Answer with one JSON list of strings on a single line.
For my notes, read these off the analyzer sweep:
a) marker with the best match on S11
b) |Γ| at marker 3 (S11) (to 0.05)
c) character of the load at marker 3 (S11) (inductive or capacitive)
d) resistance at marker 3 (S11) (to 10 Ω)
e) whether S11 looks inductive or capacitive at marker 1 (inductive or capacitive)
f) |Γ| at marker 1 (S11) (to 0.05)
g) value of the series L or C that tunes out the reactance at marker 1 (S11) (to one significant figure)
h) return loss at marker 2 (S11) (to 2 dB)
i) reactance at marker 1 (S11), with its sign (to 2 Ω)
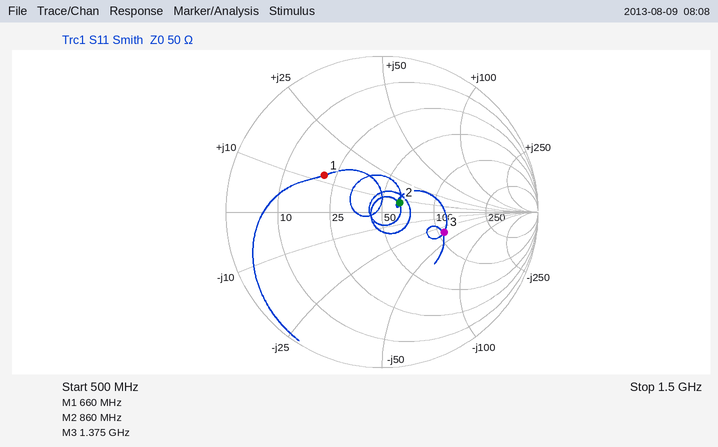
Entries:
["marker 2", "0.40", "capacitive", "110 Ω", "inductive", "0.45", "20 pF", "18 dB", "+12 Ω"]
